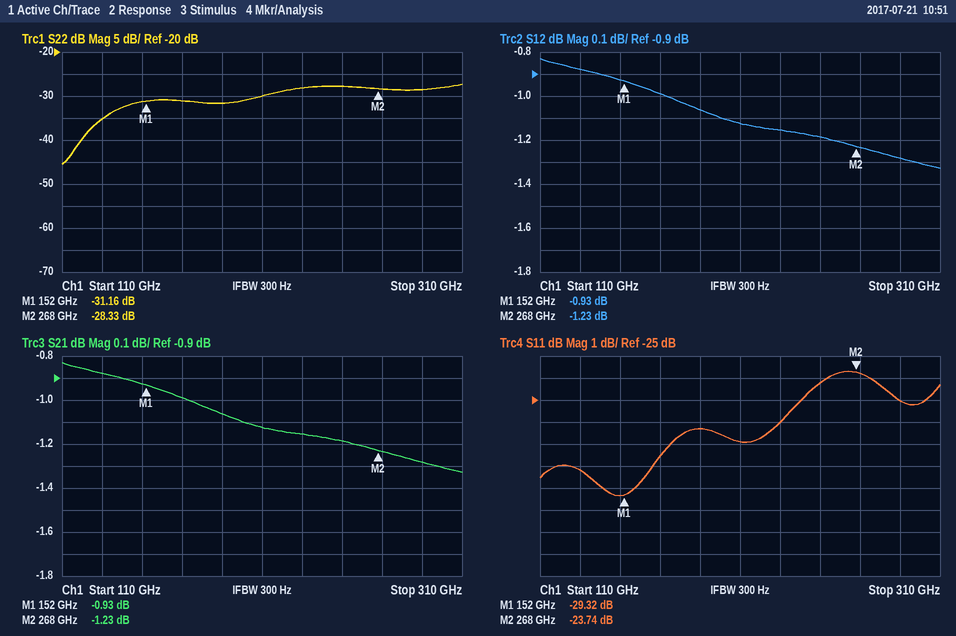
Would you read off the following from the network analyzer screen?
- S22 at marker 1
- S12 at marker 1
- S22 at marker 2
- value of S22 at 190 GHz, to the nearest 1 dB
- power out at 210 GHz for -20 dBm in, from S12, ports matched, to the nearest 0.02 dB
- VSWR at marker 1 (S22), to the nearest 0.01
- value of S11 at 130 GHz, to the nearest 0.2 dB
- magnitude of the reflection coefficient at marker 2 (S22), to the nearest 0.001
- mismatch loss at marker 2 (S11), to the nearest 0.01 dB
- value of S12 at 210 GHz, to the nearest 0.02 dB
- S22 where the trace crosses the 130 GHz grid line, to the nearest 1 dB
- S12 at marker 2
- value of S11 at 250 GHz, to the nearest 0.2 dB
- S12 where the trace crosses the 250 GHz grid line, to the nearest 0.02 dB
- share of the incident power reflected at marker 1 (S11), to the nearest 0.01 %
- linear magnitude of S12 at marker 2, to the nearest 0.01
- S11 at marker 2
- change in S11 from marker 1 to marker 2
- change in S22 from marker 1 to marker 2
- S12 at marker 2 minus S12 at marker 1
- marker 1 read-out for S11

-31.16 dB
-0.93 dB
-28.33 dB
-32 dB
-21.12 dBm
1.06
-28.2 dB
0.038
0.02 dB
-1.12 dB
-35 dB
-1.23 dB
-24.2 dB
-1.18 dB
0.12 %
0.87
-23.74 dB
5.58 dB
2.83 dB
-0.30 dB
-29.32 dB
